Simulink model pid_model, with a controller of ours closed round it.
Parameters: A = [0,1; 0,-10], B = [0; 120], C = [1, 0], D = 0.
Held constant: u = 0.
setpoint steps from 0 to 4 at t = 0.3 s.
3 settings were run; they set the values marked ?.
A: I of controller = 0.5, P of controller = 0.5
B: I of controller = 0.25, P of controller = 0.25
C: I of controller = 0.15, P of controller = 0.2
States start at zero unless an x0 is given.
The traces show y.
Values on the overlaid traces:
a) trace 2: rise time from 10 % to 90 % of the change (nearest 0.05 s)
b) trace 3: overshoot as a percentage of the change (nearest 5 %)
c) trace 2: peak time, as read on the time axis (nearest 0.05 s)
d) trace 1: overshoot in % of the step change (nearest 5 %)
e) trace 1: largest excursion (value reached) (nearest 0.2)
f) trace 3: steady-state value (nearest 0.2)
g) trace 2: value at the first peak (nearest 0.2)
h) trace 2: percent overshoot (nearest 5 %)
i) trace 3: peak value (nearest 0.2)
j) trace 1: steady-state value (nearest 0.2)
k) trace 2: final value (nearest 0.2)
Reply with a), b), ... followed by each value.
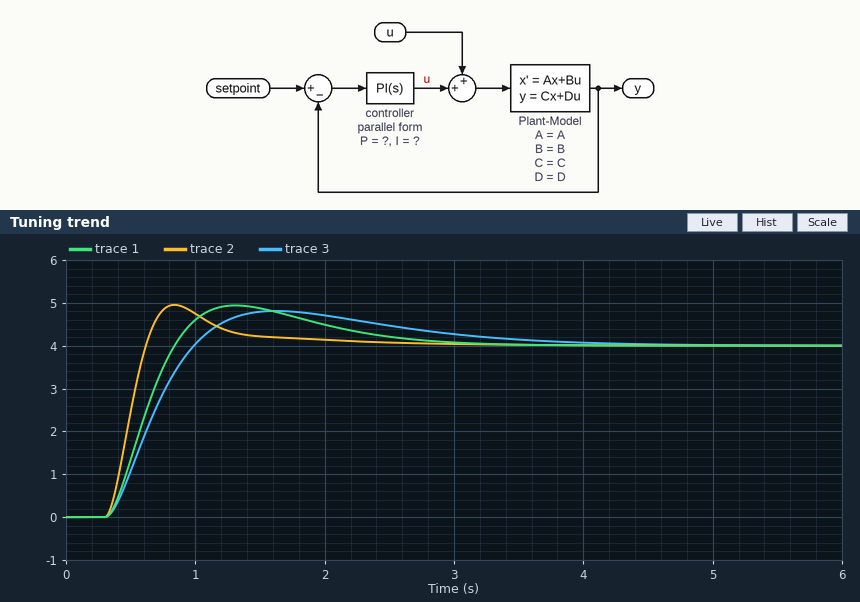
a) 0.20 s
b) 20 %
c) 0.85 s
d) 25 %
e) 5.0
f) 4.0
g) 5.0
h) 25 %
i) 4.8
j) 4.0
k) 4.0
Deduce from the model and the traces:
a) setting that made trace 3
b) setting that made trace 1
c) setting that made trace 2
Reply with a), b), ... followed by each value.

a) C
b) B
c) A
